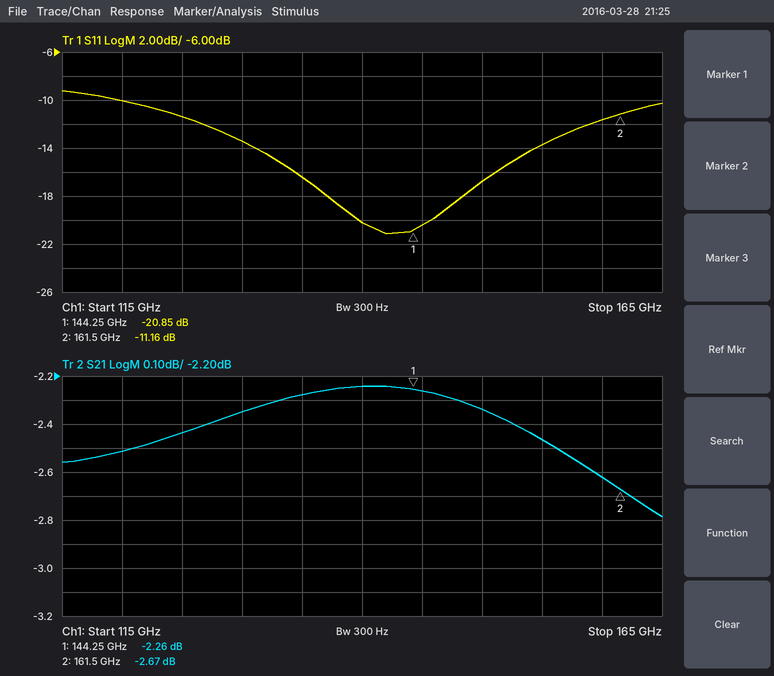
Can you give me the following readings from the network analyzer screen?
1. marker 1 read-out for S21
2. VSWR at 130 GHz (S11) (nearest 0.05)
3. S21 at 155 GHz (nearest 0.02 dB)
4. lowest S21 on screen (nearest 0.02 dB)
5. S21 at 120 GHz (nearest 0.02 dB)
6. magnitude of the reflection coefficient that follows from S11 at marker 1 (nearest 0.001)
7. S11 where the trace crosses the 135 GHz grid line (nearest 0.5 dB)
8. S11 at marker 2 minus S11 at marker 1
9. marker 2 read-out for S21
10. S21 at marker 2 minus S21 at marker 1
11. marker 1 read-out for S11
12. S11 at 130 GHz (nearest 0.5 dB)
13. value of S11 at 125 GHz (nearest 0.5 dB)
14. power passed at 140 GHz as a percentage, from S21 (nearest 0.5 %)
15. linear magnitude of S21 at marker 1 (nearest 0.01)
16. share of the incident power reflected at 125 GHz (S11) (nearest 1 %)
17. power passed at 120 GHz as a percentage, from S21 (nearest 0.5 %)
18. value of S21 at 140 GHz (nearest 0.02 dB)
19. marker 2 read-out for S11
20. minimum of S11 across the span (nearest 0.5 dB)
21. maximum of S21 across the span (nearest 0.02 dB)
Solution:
-2.26 dB
1.55
-2.46 dB
-2.78 dB
-2.52 dB
0.091
-16.5 dB
9.69 dB
-2.67 dB
-0.41 dB
-20.85 dB
-13.5 dB
-11.5 dB
59.5 %
0.77
7 %
56.0 %
-2.24 dB
-11.16 dB
-21.0 dB
-2.24 dB
